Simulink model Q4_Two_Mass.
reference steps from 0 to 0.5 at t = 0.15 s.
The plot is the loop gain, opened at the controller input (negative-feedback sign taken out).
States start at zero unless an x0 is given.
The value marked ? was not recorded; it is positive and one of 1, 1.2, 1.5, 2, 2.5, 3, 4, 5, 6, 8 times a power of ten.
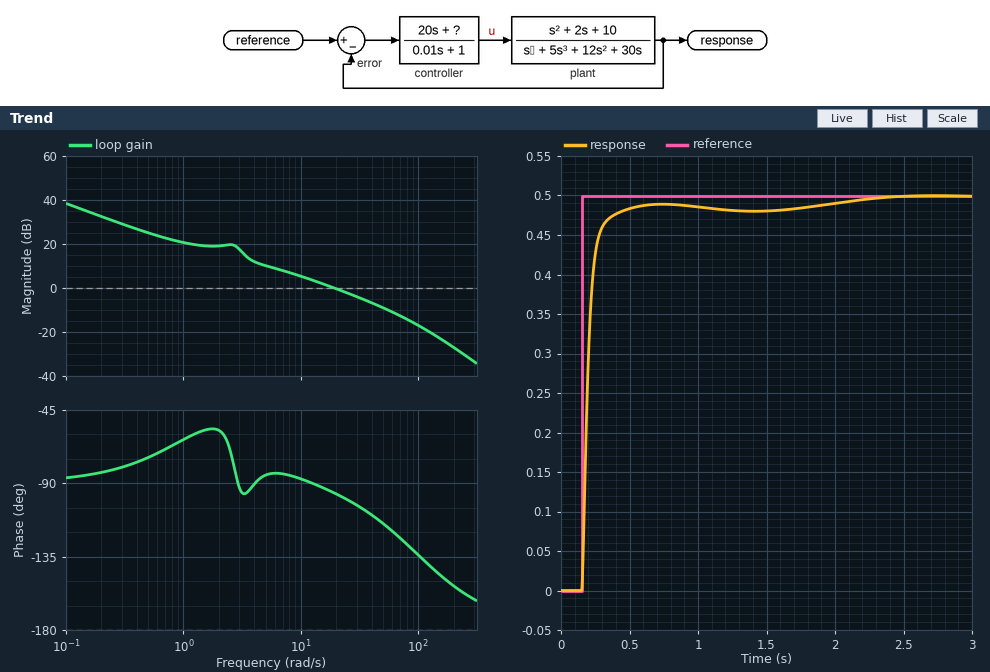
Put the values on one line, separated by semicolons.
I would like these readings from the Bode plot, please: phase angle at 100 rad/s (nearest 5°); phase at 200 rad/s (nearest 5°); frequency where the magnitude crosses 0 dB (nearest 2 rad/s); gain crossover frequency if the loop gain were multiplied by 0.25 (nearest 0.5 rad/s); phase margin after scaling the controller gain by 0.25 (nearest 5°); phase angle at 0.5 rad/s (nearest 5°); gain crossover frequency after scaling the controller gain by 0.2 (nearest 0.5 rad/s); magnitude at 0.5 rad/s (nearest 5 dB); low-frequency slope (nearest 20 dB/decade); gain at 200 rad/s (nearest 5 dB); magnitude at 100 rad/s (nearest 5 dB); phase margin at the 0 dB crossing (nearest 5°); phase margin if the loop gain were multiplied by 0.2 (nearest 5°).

-135°; -155°; 20 rad/s; 4.0 rad/s; 90°; -75°; 3.5 rad/s; 25 dB; -20 dB/decade; -25 dB; -15 dB; 85°; 85°
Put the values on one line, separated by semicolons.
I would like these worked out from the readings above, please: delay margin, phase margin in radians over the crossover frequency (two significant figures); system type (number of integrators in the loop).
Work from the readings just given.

0.074 s; 1
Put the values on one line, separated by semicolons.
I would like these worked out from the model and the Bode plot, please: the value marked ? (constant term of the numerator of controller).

25
